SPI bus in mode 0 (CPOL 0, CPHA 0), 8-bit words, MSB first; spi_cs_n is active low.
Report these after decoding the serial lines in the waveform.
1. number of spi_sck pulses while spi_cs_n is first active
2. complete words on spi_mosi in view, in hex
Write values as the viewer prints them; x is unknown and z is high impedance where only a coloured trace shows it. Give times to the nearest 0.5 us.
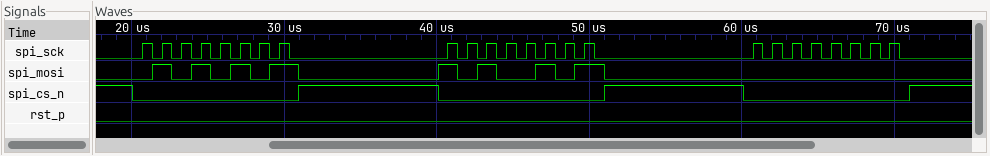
8
55, A5, 00
